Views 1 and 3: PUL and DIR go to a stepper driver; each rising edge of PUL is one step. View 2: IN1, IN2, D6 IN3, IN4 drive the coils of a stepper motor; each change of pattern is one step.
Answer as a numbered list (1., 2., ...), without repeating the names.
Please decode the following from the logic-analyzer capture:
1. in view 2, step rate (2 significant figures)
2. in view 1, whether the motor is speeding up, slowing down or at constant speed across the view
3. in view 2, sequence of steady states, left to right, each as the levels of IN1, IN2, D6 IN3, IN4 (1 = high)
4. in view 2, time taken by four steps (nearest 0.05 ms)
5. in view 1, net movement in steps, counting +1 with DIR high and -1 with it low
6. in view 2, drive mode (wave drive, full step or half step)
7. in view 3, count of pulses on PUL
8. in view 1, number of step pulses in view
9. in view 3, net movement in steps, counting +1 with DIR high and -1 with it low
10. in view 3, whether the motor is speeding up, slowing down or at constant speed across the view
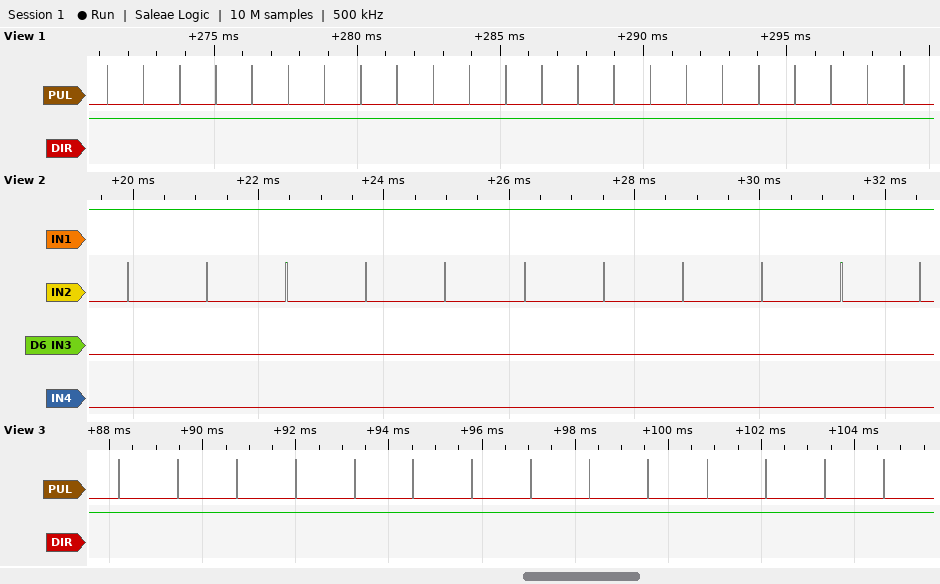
1. 790 steps/s
2. constant speed
3. 1000 1000 1000 1000 1000 1000 1000 1000 1000 1000 1000 1000
4. 5.05 ms
5. +23
6. wave drive
7. 14
8. 23
9. +14
10. constant speed
